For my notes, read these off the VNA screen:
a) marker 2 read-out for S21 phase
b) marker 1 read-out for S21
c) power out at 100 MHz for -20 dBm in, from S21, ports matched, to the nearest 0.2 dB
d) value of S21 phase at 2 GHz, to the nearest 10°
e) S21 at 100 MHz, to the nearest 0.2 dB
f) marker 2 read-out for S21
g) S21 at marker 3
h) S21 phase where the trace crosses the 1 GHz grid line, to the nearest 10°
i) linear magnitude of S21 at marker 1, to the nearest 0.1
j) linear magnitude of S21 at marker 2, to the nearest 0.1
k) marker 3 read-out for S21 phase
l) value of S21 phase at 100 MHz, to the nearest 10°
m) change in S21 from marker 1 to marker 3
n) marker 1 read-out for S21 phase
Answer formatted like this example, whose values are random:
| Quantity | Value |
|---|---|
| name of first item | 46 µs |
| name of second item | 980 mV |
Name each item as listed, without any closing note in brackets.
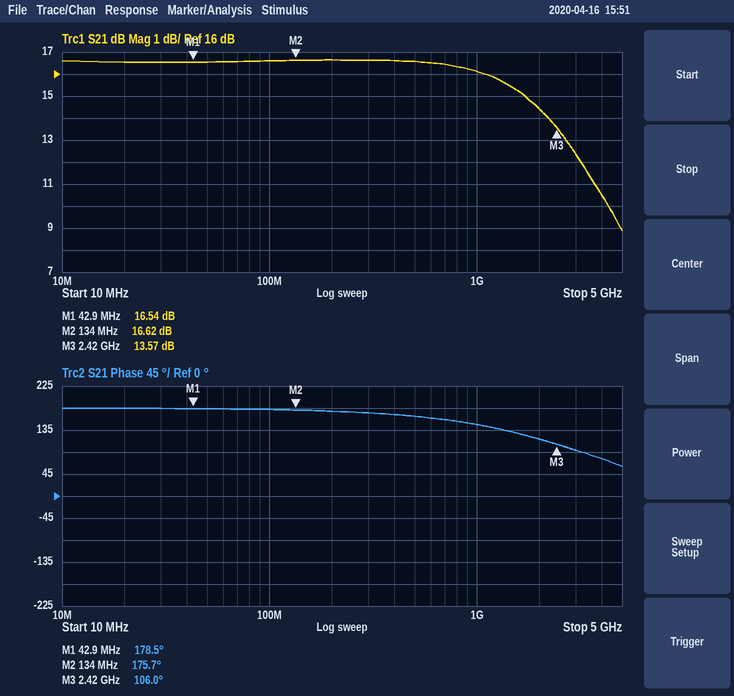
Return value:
| Quantity | Value |
|---|---|
| marker 2 read-out for S21 phase | 175.7° |
| marker 1 read-out for S21 | 16.54 dB |
| power out at 100 MHz for -20 dBm in, from S21, ports matched, to the nearest 0.2 dB | -3.4 dBm |
| value of S21 phase at 2 GHz, to the nearest 10° | 120° |
| S21 at 100 MHz, to the nearest 0.2 dB | 16.6 dB |
| marker 2 read-out for S21 | 16.62 dB |
| S21 at marker 3 | 13.57 dB |
| S21 phase where the trace crosses the 1 GHz grid line, to the nearest 10° | 150° |
| linear magnitude of S21 at marker 1, to the nearest 0.1 | 6.7 |
| linear magnitude of S21 at marker 2, to the nearest 0.1 | 6.8 |
| marker 3 read-out for S21 phase | 106.0° |
| value of S21 phase at 100 MHz, to the nearest 10° | 180° |
| change in S21 from marker 1 to marker 3 | -2.97 dB |
| marker 1 read-out for S21 phase | 178.5° |
